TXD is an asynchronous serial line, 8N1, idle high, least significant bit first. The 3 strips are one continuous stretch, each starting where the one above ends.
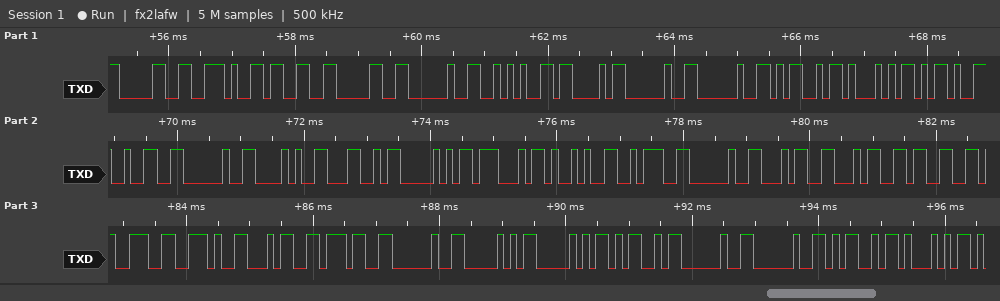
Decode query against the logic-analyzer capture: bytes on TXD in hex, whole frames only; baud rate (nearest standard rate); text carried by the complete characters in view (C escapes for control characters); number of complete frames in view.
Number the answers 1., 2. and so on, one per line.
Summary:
1. 0x30 0x2E 0x33 0x30 0x20 0x2A 0x43 0x20 0x20 0x4D 0x51 0x2D 0x32 0x20 0x28 0x4C 0x50 0x47 0x29 0x3A 0x20 0x34 0x34 0x33 0x39 0x2E 0x34 0x37 0x20 0x50 0x50 0x4D 0x20 0x20 0x4D 0x51
2. 9600 baud
3. "0.30 *C  MQ-2 (LPG): 4439.47 PPM  MQ"
4. 36
